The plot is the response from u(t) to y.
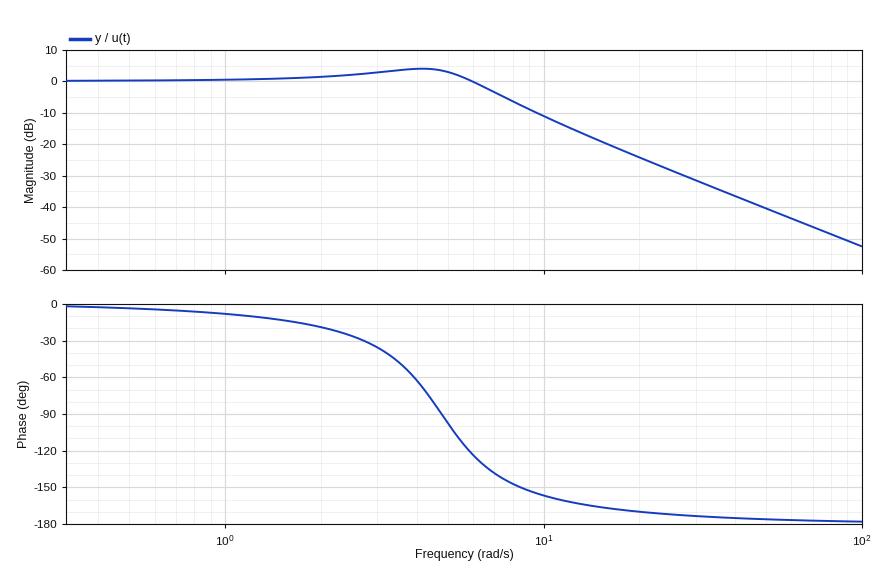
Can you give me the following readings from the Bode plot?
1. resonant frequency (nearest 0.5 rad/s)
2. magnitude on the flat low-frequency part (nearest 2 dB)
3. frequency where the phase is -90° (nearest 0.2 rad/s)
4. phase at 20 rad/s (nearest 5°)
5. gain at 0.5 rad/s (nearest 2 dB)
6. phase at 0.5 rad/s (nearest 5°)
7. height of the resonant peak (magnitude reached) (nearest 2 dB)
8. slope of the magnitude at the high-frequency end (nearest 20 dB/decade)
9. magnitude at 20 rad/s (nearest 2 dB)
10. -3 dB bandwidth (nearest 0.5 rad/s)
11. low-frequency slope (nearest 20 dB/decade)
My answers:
4.0 rad/s
0 dB
4.8 rad/s
-170°
0 dB
-5°
4 dB
-40 dB/decade
-24 dB
7.0 rad/s
0 dB/decade
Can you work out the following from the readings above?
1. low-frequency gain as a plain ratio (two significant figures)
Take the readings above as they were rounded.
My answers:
1.0
